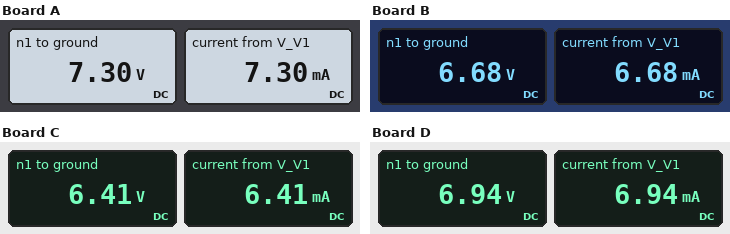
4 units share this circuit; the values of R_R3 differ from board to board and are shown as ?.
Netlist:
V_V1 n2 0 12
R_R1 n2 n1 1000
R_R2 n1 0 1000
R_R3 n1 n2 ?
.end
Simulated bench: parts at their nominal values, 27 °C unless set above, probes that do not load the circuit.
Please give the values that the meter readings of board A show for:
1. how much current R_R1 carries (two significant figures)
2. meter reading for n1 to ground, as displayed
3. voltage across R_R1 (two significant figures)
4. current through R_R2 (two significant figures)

4.7 mA
7.30 V
4.7 V
7.3 mA
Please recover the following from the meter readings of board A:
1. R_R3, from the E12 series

1.8 kΩ
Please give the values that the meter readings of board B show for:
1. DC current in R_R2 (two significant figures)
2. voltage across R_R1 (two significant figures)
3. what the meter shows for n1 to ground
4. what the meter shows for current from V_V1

6.7 mA
5.3 V
6.68 V
6.68 mA
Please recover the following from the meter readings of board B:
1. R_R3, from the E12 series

3.9 kΩ
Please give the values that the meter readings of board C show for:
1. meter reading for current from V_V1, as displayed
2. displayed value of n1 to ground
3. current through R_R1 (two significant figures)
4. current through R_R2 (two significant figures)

6.41 mA
6.41 V
5.6 mA
6.4 mA
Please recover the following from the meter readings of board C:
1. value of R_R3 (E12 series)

6.8 kΩ
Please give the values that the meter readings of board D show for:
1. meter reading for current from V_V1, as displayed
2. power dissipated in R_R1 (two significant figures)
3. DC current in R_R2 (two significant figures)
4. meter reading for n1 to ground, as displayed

6.94 mA
26 mW
6.9 mA
6.94 V
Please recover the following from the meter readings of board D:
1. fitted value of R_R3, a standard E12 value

2.7 kΩ
